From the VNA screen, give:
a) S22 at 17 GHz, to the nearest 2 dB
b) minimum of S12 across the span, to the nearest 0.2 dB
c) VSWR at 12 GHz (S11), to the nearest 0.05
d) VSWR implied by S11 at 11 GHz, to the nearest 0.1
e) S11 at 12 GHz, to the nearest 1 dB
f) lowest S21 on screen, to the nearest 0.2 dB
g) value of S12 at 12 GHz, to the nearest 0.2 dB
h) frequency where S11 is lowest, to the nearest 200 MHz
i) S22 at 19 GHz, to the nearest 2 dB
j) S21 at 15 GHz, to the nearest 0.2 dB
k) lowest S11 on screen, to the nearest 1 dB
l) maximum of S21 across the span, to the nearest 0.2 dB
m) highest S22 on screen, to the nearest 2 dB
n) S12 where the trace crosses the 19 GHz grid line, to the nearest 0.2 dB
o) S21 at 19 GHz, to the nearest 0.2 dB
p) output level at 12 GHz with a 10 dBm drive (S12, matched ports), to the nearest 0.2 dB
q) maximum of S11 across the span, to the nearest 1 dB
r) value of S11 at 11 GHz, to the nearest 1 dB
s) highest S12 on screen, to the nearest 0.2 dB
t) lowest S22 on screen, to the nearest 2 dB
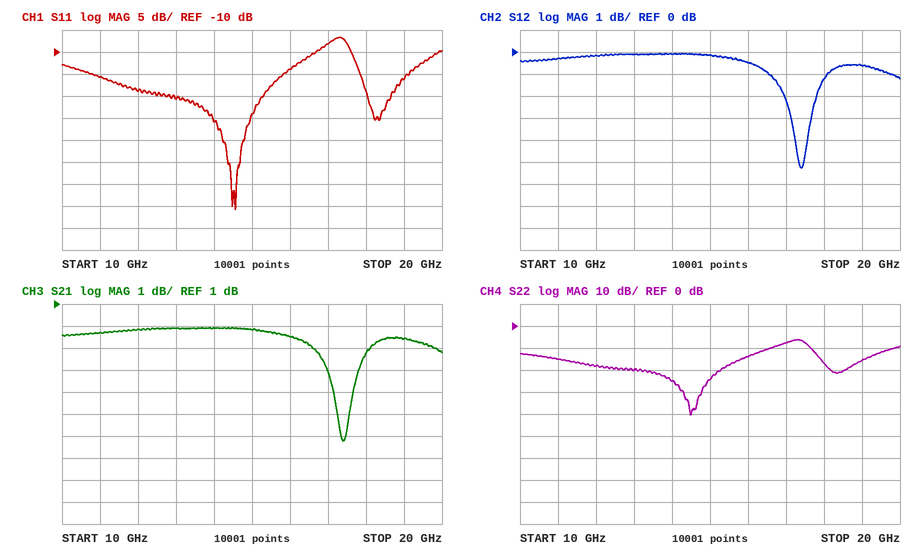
-8 dB
-5.2 dB
1.25
1.4
-19 dB
-5.2 dB
-0.2 dB
14.6 GHz
-16 dB
-0.2 dB
-46 dB
0.0 dB
-6 dB
-0.6 dB
-0.6 dB
9.8 dBm
-7 dB
-16 dB
0.0 dB
-40 dB
